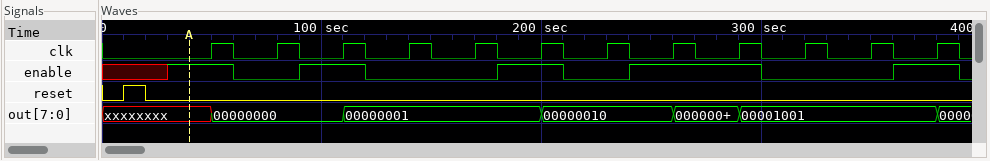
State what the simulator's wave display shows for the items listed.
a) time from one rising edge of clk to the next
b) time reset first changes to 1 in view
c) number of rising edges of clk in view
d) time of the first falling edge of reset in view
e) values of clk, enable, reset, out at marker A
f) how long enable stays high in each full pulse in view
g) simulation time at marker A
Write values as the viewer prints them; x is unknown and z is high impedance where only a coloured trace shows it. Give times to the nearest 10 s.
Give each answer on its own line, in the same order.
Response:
30 s
10 s
12
20 s
clk=0, enable=1, reset=0, out=xxxxxxxx
30 s, 30 s, 60 s, 30 s
40 s
